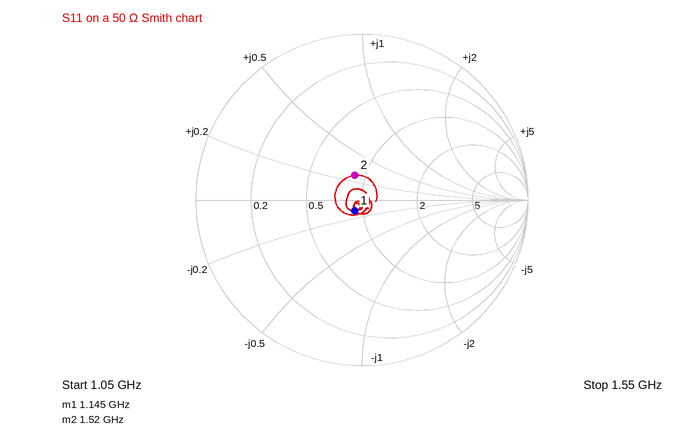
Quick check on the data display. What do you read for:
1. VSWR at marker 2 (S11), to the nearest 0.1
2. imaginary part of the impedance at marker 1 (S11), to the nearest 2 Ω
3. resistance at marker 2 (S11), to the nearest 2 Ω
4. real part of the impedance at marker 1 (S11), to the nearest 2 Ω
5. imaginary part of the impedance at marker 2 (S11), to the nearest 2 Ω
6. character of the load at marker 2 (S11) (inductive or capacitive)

1.4
-6 Ω
44 Ω
46 Ω
+14 Ω
inductive
